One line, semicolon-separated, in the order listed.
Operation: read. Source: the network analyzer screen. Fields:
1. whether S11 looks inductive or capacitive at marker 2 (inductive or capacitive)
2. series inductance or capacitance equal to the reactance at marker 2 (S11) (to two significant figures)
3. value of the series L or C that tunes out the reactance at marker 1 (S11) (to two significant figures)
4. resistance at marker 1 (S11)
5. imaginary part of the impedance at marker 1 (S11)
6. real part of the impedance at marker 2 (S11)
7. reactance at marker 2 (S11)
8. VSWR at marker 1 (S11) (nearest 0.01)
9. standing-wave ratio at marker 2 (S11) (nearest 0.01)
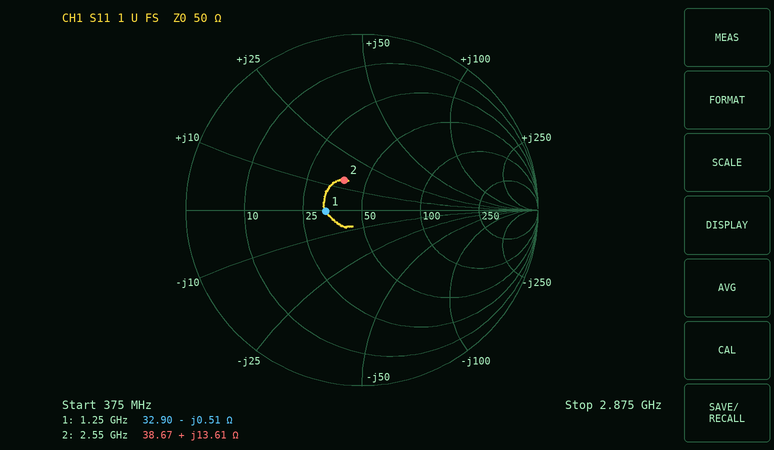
inductive; 850 pH; 65 pH; 32.90 Ω; -0.51 Ω; 38.67 Ω; +13.61 Ω; 1.52; 1.49
